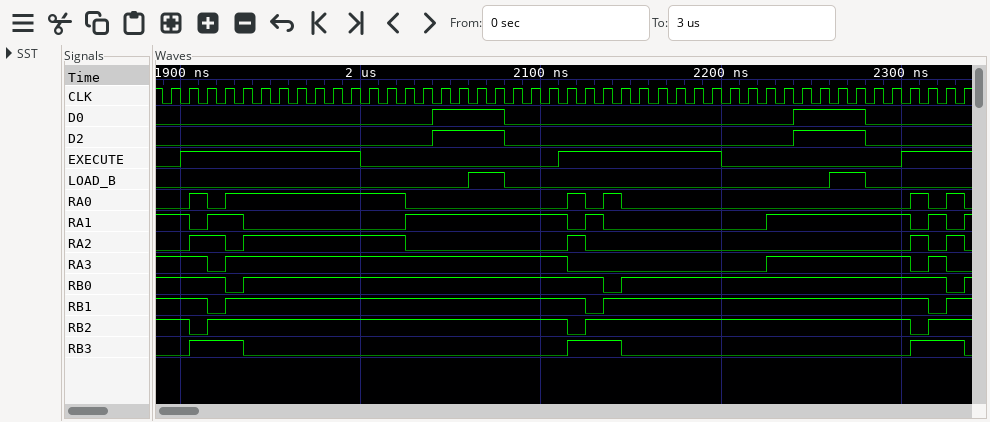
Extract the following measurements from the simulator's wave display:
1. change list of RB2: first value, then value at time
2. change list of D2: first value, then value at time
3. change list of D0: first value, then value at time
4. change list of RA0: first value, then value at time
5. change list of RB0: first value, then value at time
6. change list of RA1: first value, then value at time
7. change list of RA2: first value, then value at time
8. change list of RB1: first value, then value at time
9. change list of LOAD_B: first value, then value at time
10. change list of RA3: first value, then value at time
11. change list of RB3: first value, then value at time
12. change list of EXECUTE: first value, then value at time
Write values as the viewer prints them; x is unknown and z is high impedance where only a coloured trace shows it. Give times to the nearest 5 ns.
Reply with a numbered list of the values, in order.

1. 1, 0 at 1905 ns, 1 at 1915 ns, 0 at 2115 ns, 1 at 2125 ns, 0 at 2305 ns, 1 at 2315 ns
2. 0, 1 at 2040 ns, 0 at 2080 ns, 1 at 2240 ns, 0 at 2280 ns
3. 0, 1 at 2040 ns, 0 at 2080 ns, 1 at 2240 ns, 0 at 2280 ns
4. 0, 1 at 1905 ns, 0 at 1915 ns, 1 at 1925 ns, 0 at 2025 ns, 1 at 2115 ns, 0 at 2125 ns, 1 at 2135 ns, 0 at 2145 ns, 1 at 2305 ns, 0 at 2315 ns, 1 at 2325 ns, 0 at 2335 ns
5. 1, 0 at 1925 ns, 1 at 1935 ns, 0 at 2135 ns, 1 at 2145 ns, 0 at 2325 ns, 1 at 2335 ns
6. 1, 0 at 1905 ns, 1 at 1915 ns, 0 at 1935 ns, 1 at 2025 ns, 0 at 2115 ns, 1 at 2125 ns, 0 at 2135 ns, 1 at 2225 ns, 0 at 2305 ns, 1 at 2315 ns, 0 at 2325 ns, 1 at 2335 ns
7. 0, 1 at 1905 ns, 0 at 1925 ns, 1 at 1935 ns, 0 at 2025 ns, 1 at 2115 ns, 0 at 2125 ns, 1 at 2305 ns, 0 at 2315 ns, 1 at 2325 ns, 0 at 2335 ns
8. 1, 0 at 1915 ns, 1 at 1925 ns, 0 at 2125 ns, 1 at 2135 ns, 0 at 2315 ns, 1 at 2325 ns
9. 0, 1 at 2060 ns, 0 at 2080 ns, 1 at 2260 ns, 0 at 2280 ns
10. 1, 0 at 1915 ns, 1 at 1925 ns, 0 at 2115 ns, 1 at 2225 ns, 0 at 2305 ns, 1 at 2315 ns, 0 at 2325 ns
11. 0, 1 at 1905 ns, 0 at 1935 ns, 1 at 2115 ns, 0 at 2145 ns, 1 at 2305 ns, 0 at 2335 ns
12. 0, 1 at 1900 ns, 0 at 2000 ns, 1 at 2110 ns, 0 at 2200 ns, 1 at 2300 ns
